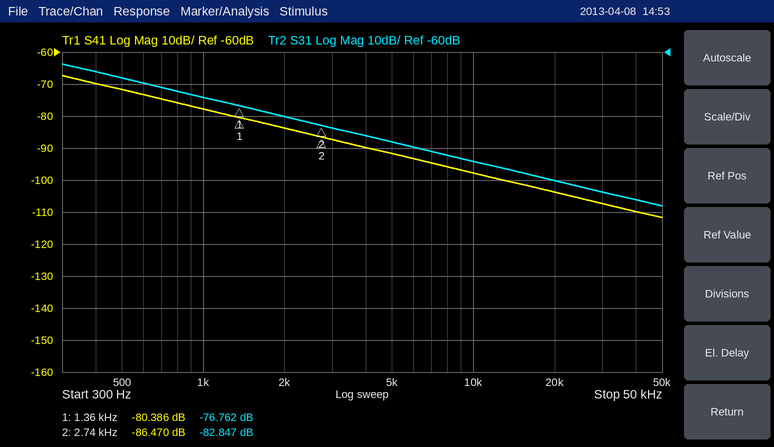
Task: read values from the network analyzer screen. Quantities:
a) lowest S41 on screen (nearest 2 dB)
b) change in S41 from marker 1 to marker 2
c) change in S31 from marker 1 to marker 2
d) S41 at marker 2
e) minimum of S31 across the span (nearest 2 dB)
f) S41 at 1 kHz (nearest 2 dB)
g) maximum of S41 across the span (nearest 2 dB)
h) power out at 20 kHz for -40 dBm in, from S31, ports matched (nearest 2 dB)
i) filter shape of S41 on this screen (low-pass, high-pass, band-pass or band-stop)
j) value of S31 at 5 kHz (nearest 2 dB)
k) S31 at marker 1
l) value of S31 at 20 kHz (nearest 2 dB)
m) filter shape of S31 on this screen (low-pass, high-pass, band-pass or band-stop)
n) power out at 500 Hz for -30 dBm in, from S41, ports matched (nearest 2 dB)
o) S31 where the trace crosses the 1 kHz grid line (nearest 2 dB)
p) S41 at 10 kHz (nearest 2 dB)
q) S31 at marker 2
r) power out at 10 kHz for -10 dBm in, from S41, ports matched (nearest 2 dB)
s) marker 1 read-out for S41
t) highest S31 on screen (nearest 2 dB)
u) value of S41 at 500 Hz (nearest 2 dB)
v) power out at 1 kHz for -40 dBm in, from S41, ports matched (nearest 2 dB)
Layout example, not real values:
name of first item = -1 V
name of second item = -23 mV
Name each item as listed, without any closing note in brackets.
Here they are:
lowest S41 on screen = -112 dB
change in S41 from marker 1 to marker 2 = -6.084 dB
change in S31 from marker 1 to marker 2 = -6.085 dB
S41 at marker 2 = -86.470 dB
minimum of S31 across the span = -108 dB
S41 at 1 kHz = -78 dB
maximum of S41 across the span = -68 dB
power out at 20 kHz for -40 dBm in, from S31, ports matched = -140 dBm
filter shape of S41 on this screen = low-pass
value of S31 at 5 kHz = -88 dB
S31 at marker 1 = -76.762 dB
value of S31 at 20 kHz = -100 dB
filter shape of S31 on this screen = low-pass
power out at 500 Hz for -30 dBm in, from S41, ports matched = -102 dBm
S31 where the trace crosses the 1 kHz grid line = -74 dB
S41 at 10 kHz = -98 dB
S31 at marker 2 = -82.847 dB
power out at 10 kHz for -10 dBm in, from S41, ports matched = -108 dBm
marker 1 read-out for S41 = -80.386 dB
highest S31 on screen = -64 dB
value of S41 at 500 Hz = -72 dB
power out at 1 kHz for -40 dBm in, from S41, ports matched = -118 dBm
